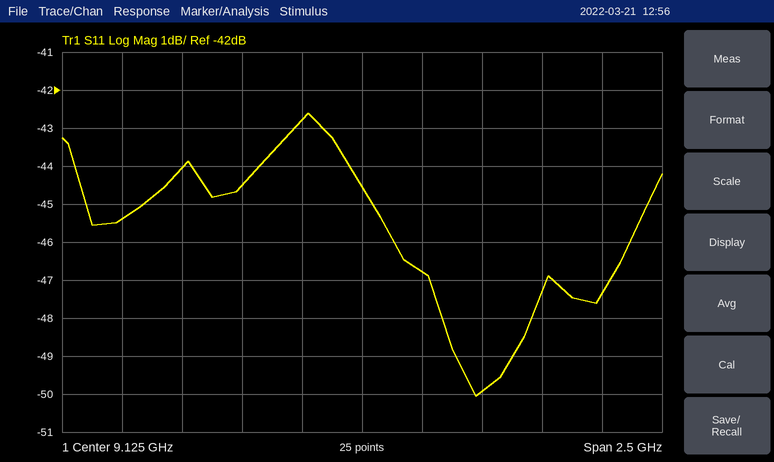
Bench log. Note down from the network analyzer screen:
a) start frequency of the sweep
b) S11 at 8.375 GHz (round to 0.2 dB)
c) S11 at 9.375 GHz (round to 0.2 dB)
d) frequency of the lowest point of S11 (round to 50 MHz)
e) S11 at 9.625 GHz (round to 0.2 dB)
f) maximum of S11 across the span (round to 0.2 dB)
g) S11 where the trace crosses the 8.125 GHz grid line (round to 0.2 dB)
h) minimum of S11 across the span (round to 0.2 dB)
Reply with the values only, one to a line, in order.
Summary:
7.875 GHz
-44.0 dB
-46.8 dB
9.60 GHz
-50.0 dB
-42.6 dB
-45.4 dB
-50.0 dB
